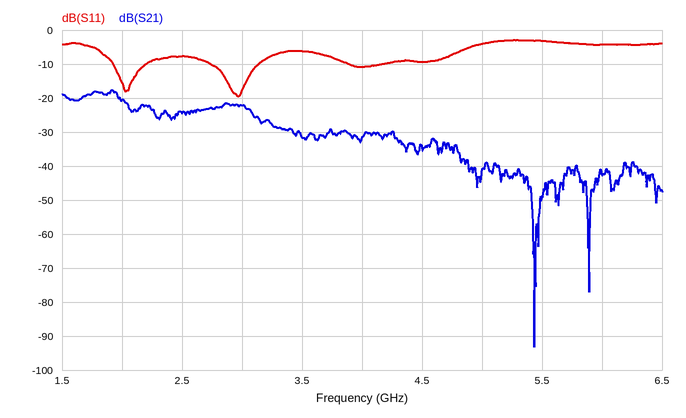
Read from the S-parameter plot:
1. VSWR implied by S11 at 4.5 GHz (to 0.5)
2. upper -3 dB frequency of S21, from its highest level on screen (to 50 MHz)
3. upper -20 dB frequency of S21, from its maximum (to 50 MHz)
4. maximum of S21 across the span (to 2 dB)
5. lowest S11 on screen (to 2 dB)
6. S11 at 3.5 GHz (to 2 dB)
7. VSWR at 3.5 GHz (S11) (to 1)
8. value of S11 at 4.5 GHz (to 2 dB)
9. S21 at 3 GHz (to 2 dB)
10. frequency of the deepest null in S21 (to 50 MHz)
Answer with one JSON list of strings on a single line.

["2.0", "2.00 GHz", "4.80 GHz", "-18 dB", "-20 dB", "-6 dB", "3", "-10 dB", "-22 dB", "5.45 GHz"]
